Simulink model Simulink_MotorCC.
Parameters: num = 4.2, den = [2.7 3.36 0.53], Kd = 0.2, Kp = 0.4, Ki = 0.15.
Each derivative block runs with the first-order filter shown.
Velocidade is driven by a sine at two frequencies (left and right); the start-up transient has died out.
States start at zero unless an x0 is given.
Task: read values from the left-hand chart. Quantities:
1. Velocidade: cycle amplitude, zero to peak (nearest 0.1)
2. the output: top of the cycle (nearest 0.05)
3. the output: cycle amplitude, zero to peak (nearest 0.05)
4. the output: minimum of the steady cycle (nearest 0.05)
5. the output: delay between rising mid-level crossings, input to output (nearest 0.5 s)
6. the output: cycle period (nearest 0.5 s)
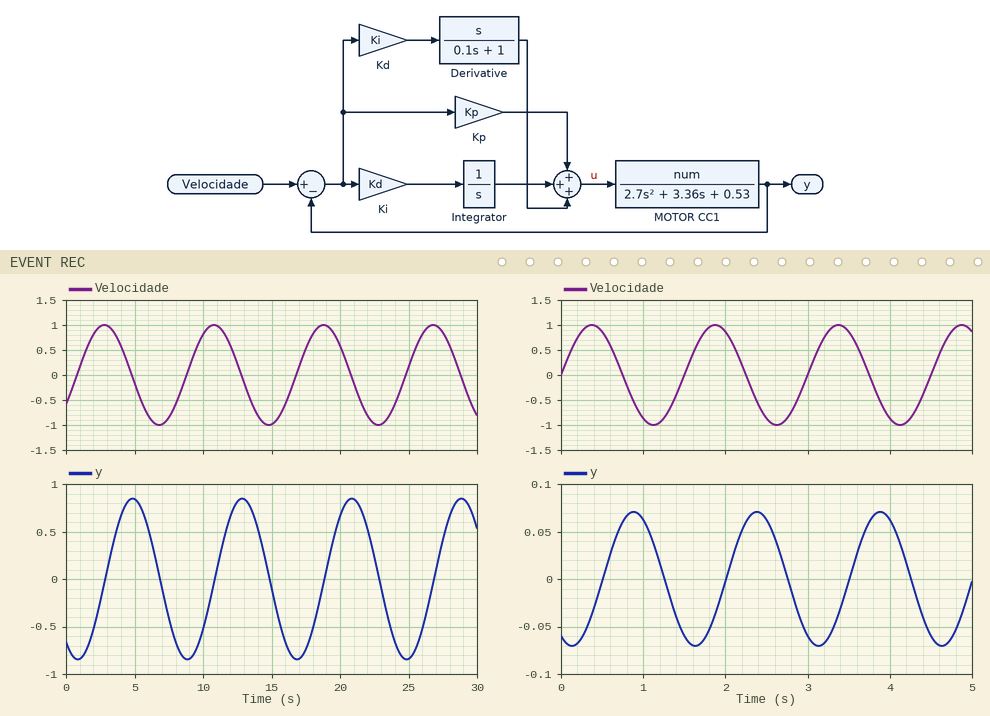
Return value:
1.0
0.85
0.85
-0.85
2.0 s
8.0 s
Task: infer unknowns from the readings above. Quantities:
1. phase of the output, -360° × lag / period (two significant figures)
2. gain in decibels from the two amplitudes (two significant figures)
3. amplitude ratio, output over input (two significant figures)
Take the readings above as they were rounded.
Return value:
-90°
-1.4 dB
0.85
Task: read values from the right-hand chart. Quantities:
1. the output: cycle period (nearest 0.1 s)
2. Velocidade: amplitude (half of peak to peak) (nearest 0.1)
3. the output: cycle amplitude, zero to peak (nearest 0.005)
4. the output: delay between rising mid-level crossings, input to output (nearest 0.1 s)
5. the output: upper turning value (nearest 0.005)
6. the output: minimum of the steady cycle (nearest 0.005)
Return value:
1.5 s
1.0
0.070
0.5 s
0.070
-0.070
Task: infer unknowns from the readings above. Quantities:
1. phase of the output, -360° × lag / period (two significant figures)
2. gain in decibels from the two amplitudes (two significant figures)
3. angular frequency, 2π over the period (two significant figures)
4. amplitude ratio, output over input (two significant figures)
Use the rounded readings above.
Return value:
-120°
-23 dB
4.2 rad/s
0.070
